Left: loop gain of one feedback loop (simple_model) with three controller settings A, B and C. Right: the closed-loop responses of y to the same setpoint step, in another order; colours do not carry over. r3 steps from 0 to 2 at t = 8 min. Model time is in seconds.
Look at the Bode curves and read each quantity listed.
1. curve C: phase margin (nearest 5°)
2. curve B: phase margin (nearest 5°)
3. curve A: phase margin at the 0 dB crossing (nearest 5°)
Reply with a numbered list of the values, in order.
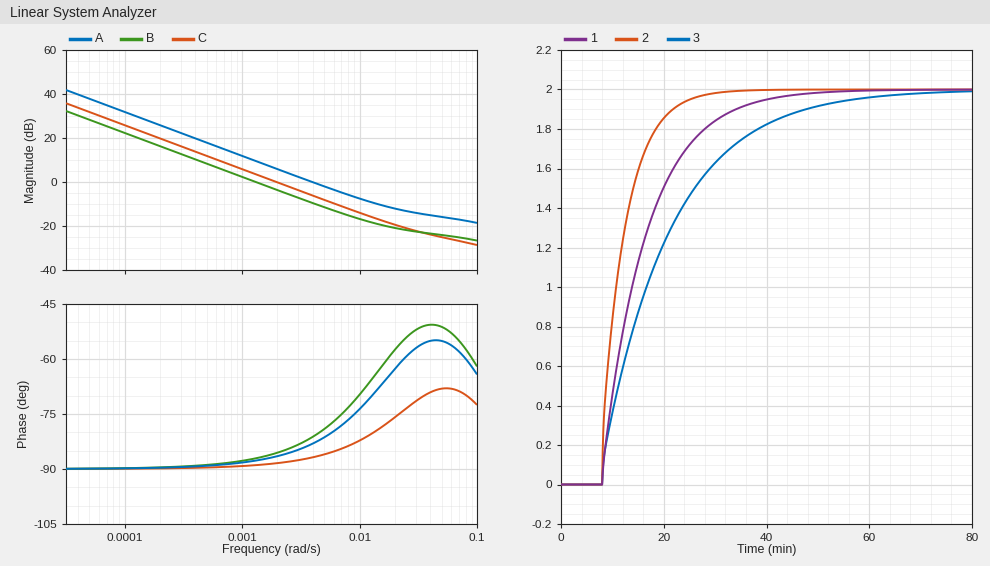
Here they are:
1. 90°
2. 95°
3. 95°
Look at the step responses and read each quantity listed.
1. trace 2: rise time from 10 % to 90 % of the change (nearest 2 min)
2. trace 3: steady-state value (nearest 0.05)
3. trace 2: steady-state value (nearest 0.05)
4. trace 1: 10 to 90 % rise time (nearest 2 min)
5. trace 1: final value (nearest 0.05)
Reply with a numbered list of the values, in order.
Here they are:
1. 10 min
2. 2.00
3. 2.00
4. 20 min
5. 2.00
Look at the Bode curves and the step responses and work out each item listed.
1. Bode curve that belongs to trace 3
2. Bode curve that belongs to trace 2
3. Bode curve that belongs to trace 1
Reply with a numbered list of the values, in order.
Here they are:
1. B
2. A
3. C
